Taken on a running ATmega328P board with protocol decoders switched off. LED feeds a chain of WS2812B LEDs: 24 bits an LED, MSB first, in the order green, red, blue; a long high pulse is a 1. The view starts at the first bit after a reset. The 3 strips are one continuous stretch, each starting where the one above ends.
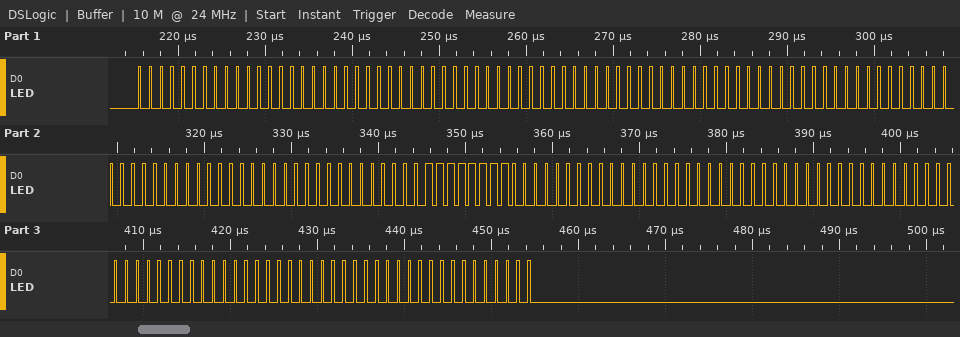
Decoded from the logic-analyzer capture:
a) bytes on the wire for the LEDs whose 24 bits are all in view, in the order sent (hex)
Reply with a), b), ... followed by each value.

a) 00 00 00 00 00 00 00 00 00 00 00 00 00 FF 00 00 00 00 00 00 00 00 00 00
